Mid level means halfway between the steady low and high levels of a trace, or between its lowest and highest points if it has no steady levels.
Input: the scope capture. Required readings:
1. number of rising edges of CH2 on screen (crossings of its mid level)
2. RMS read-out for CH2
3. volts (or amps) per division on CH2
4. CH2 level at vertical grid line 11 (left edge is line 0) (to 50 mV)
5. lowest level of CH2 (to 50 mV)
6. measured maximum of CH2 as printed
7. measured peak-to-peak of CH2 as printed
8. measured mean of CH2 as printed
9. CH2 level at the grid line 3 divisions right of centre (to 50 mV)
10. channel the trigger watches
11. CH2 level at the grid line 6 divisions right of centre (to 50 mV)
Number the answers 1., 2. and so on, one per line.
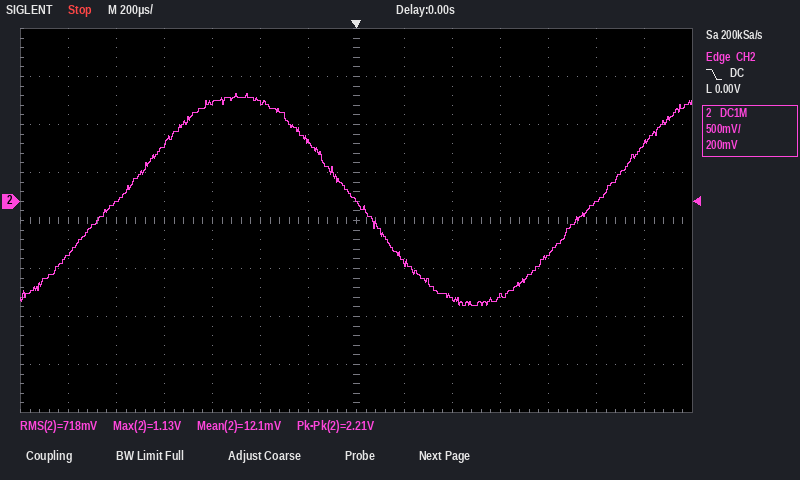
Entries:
1. 2
2. 718 mV
3. 500 mV
4. -550 mV
5. -1.10 V
6. 1.13 V
7. 2.21 V
8. 12.1 mV
9. -1.00 V
10. CH2
11. 600 mV
